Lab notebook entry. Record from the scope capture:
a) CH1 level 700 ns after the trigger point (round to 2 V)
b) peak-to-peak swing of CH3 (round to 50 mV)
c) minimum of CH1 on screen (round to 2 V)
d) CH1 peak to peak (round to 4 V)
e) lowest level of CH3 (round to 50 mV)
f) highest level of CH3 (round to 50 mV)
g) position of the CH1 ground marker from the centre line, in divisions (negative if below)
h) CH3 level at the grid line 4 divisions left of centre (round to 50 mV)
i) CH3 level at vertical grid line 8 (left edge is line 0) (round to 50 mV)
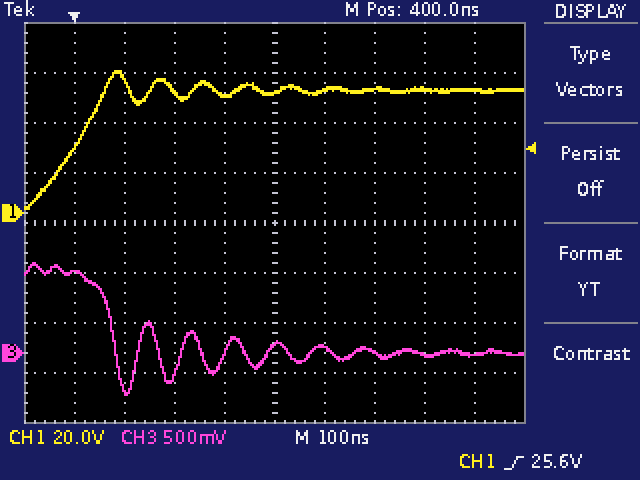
50 V
1.30 V
2 V
56 V
-400 mV
900 mV
+0.2 div
800 mV
0 mV
